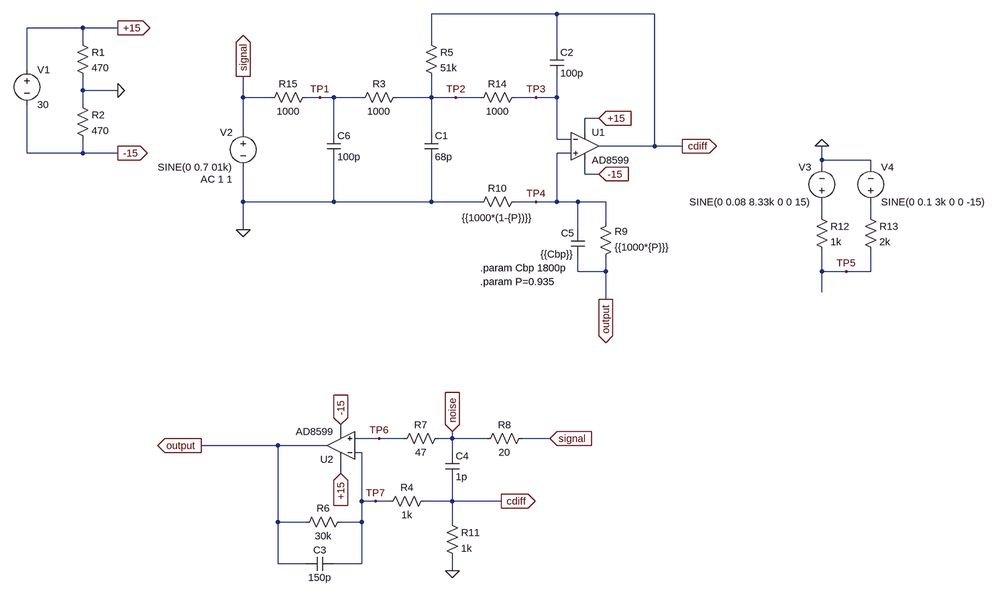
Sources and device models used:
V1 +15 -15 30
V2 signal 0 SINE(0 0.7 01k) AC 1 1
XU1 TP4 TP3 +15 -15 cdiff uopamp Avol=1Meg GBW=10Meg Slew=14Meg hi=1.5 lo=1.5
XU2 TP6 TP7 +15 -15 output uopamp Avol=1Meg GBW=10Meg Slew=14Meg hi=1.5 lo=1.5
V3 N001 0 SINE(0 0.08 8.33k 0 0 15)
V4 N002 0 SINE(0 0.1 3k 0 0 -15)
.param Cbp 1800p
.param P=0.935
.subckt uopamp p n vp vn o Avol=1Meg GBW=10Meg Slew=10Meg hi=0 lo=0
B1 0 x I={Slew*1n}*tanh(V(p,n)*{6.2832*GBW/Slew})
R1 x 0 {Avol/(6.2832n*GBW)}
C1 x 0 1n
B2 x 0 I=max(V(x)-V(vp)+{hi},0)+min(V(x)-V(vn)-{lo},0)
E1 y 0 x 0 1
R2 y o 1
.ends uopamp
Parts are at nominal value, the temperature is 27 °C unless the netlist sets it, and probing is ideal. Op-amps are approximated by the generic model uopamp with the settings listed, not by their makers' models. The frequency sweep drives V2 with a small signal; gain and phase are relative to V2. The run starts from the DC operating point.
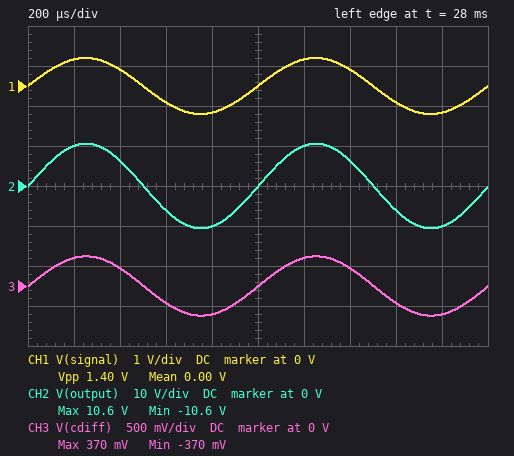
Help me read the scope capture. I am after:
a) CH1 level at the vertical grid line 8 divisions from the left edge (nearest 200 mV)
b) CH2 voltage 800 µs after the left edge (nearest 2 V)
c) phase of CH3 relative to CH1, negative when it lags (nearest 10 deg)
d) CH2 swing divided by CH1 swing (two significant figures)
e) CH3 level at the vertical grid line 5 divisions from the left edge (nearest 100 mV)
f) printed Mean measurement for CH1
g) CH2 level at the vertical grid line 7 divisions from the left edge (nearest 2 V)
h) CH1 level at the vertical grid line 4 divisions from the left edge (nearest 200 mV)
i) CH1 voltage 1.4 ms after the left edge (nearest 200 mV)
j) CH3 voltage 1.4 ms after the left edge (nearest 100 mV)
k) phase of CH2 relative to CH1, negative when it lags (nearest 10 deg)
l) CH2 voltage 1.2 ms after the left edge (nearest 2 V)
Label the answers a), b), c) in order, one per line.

a) -400 mV
b) -10 V
c) 0 deg
d) 15
e) 0 V
f) 0.00 V
g) 6 V
h) -600 mV
i) 400 mV
j) 200 mV
k) 0 deg
l) 10 V
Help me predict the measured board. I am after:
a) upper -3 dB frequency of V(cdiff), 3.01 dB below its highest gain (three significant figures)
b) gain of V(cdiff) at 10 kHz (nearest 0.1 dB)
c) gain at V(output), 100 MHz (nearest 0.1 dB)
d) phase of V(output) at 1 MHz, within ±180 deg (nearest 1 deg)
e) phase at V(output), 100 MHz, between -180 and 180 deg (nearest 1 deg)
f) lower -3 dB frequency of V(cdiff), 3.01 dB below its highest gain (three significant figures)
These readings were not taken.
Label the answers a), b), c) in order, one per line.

a) 6.00 MHz
b) -5.6 dB
c) -20.2 dB
d) -20 deg
e) -85 deg
f) 572 kHz
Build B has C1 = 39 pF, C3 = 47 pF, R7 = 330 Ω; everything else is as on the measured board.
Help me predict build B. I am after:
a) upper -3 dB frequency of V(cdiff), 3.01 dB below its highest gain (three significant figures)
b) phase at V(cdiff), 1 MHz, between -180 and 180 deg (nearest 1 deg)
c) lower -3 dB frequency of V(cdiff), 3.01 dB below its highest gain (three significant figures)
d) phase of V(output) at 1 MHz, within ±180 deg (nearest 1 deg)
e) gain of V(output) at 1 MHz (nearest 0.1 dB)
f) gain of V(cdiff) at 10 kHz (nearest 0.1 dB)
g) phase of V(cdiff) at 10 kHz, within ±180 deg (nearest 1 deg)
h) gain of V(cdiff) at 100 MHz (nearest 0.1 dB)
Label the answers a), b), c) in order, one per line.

a) 7.02 MHz
b) 5 deg
c) 589 kHz
d) -45 deg
e) -1.8 dB
f) -5.5 dB
g) 0 deg
h) -40.3 dB
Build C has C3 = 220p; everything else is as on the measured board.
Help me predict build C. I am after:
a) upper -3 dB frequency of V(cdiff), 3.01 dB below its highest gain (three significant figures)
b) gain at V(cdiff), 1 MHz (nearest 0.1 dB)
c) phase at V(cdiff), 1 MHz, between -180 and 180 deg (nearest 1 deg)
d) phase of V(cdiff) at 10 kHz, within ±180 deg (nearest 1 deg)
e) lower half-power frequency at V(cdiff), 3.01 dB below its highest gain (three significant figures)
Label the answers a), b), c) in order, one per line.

a) 5.83 MHz
b) -0.7 dB
c) 21 deg
d) -16 deg
e) 352 kHz
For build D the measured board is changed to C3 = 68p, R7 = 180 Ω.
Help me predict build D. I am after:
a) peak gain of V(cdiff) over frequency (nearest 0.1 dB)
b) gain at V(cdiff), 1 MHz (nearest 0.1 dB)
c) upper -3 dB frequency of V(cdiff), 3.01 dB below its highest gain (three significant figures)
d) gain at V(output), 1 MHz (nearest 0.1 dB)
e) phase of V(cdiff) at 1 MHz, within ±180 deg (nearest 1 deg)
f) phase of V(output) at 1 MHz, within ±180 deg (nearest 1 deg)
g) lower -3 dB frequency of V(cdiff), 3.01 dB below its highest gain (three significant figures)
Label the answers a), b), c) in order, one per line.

a) 0.5 dB
b) -1.6 dB
c) 6.38 MHz
d) -3.1 dB
e) 8 deg
f) -36 deg
g) 636 kHz
